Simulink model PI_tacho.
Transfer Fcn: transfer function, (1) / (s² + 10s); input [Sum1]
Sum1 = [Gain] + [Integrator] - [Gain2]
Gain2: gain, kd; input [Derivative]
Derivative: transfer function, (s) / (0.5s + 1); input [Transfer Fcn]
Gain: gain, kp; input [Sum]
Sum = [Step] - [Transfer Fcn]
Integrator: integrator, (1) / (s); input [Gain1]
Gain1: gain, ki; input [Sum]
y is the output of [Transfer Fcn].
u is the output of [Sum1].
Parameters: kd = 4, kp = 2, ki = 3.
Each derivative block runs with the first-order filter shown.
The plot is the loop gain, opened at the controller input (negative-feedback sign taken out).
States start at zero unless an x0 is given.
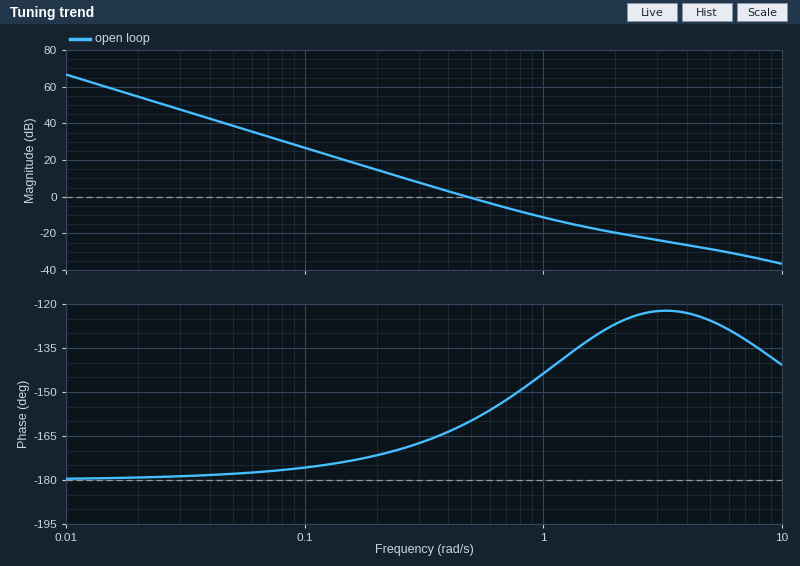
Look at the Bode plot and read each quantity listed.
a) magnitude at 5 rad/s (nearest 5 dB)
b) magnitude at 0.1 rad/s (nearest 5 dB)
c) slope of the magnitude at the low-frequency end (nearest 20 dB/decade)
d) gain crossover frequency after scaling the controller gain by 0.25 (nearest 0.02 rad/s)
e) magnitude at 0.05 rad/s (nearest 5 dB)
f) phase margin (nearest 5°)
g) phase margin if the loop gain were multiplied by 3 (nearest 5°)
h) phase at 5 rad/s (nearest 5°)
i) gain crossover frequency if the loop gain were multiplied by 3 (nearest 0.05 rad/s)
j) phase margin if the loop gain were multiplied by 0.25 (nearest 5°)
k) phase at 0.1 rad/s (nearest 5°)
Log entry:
-30 dB
25 dB
-40 dB/decade
0.24 rad/s
40 dB
20°
35°
-125°
0.90 rad/s
10°
-175°
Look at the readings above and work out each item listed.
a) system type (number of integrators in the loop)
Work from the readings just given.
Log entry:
2
